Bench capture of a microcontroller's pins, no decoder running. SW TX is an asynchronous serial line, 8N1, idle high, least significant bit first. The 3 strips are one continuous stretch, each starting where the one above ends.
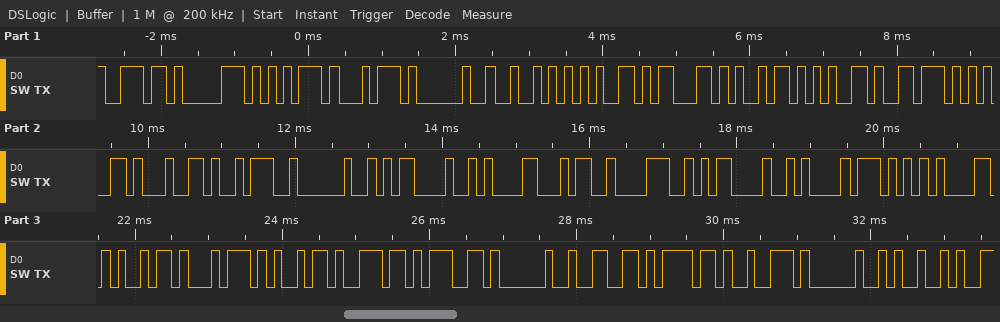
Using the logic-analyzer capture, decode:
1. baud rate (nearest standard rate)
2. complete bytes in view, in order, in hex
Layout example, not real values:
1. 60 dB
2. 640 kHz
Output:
1. 9600 baud
2. 6E 70 75 74 20 52 65 63 69 65 76 65 64 3A 20 0D 0A 34 38 0D 0A 57 61 69 74 69 6E 67 20 66 6F 72 20 49
